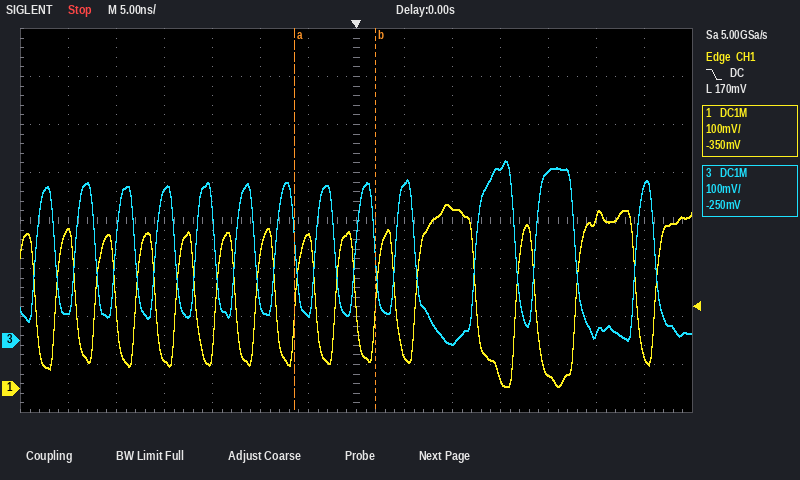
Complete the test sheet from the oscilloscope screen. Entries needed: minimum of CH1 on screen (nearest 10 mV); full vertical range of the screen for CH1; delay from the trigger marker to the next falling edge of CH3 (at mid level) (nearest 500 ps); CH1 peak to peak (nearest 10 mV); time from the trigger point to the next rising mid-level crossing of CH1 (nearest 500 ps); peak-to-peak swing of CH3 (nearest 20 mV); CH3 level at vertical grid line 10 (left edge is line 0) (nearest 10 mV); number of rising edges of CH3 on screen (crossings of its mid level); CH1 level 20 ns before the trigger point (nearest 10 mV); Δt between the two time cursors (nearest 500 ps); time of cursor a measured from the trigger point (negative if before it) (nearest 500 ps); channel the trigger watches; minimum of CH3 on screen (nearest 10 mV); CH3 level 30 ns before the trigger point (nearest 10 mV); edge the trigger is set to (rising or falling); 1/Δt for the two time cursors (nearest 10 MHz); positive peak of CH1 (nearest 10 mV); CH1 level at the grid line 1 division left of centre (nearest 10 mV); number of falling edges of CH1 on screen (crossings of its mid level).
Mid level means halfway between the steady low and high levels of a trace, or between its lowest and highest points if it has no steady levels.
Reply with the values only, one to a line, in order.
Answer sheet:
0 mV
800 mV
2.0 ns
380 mV
2.0 ns
380 mV
360 mV
13
60 mV
8.5 ns
-6.5 ns
CH1
-10 mV
60 mV
falling
120 MHz
380 mV
320 mV
13
